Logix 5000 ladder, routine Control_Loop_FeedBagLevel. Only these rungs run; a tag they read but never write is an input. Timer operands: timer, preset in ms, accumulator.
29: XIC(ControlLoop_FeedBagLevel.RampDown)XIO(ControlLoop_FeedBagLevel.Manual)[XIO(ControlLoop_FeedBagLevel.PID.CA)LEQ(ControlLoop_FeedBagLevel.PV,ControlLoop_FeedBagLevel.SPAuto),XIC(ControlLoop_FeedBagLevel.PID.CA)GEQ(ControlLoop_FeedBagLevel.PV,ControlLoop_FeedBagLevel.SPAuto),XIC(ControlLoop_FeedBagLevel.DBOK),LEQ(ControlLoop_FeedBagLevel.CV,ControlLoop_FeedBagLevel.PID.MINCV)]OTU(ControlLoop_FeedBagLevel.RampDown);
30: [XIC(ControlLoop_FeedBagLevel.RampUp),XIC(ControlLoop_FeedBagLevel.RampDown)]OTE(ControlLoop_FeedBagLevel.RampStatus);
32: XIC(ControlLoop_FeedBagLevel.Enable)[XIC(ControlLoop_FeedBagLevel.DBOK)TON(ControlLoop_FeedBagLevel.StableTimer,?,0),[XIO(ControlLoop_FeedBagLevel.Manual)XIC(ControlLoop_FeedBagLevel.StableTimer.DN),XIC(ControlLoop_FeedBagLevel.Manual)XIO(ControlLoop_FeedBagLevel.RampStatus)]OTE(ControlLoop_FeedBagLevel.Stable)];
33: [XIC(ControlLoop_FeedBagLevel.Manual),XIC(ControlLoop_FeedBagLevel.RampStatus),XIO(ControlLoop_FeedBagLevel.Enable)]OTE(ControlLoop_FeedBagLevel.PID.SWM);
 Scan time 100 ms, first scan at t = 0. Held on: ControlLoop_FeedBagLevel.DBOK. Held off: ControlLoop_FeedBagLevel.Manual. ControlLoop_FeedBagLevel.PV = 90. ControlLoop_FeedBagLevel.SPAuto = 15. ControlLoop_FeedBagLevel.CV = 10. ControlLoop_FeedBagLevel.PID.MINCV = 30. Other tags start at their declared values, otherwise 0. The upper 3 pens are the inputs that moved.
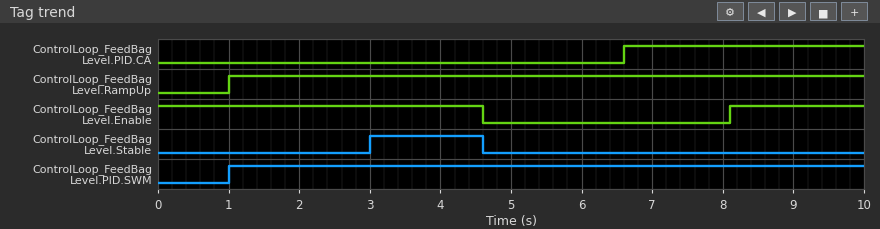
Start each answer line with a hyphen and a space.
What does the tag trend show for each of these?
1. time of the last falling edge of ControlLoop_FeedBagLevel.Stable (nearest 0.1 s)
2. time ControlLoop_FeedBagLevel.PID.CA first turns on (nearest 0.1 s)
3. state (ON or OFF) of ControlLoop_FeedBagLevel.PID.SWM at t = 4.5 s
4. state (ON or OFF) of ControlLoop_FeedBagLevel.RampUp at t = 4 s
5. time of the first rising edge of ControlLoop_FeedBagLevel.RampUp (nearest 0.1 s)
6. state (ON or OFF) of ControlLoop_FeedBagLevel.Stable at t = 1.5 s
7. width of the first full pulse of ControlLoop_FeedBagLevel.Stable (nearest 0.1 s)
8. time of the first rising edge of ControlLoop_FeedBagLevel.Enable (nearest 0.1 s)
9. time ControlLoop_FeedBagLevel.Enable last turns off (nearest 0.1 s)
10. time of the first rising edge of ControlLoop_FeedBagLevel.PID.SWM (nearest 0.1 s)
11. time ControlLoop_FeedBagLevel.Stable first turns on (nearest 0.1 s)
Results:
- 4.6 s
- 6.6 s
- ON
- ON
- 1.0 s
- OFF
- 1.6 s
- 8.1 s
- 4.6 s
- 1.0 s
- 3.0 s
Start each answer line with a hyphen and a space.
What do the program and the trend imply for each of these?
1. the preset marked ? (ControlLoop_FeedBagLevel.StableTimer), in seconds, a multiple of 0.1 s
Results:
- 3.0 s
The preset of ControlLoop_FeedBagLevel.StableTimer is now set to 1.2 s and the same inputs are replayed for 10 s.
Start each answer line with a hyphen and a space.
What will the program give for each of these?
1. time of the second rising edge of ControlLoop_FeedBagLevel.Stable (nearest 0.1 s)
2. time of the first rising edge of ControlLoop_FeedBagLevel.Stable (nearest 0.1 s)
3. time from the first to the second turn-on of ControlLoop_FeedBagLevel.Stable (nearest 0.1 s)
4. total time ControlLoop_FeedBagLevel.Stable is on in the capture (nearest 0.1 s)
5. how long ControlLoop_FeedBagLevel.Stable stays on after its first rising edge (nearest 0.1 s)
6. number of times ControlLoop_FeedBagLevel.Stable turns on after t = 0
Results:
- 9.3 s
- 1.2 s
- 8.1 s
- 4.1 s
- 3.4 s
- 2
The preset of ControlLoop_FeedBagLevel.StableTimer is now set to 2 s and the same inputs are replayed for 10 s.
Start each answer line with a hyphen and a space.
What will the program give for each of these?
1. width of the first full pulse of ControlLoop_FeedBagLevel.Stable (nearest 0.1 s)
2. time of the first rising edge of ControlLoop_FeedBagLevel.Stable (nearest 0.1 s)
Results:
- 2.6 s
- 2.0 s
